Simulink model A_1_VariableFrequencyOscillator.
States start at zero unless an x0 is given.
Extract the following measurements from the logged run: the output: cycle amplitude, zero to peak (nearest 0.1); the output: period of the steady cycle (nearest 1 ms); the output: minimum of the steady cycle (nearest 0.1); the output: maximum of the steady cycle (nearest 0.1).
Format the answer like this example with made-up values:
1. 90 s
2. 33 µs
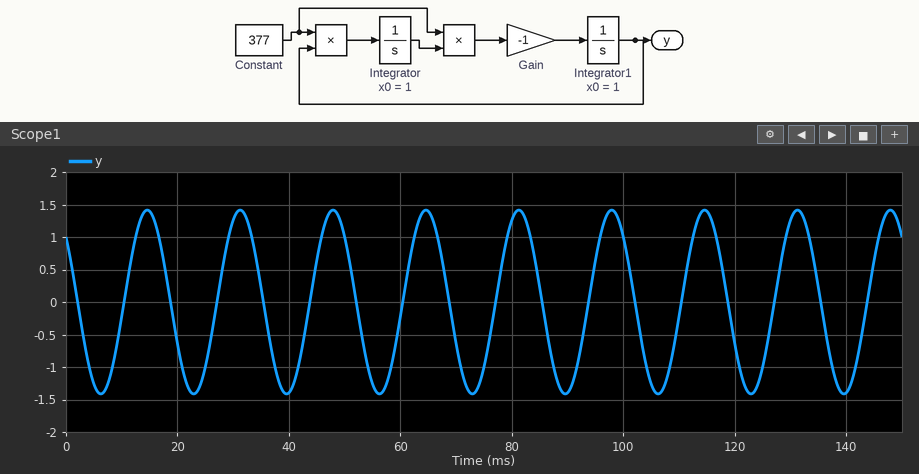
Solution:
1. 1.4
2. 17 ms
3. -1.4
4. 1.4
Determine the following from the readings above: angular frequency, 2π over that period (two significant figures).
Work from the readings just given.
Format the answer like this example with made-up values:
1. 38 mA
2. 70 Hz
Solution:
1. 0.37 rad/ms
